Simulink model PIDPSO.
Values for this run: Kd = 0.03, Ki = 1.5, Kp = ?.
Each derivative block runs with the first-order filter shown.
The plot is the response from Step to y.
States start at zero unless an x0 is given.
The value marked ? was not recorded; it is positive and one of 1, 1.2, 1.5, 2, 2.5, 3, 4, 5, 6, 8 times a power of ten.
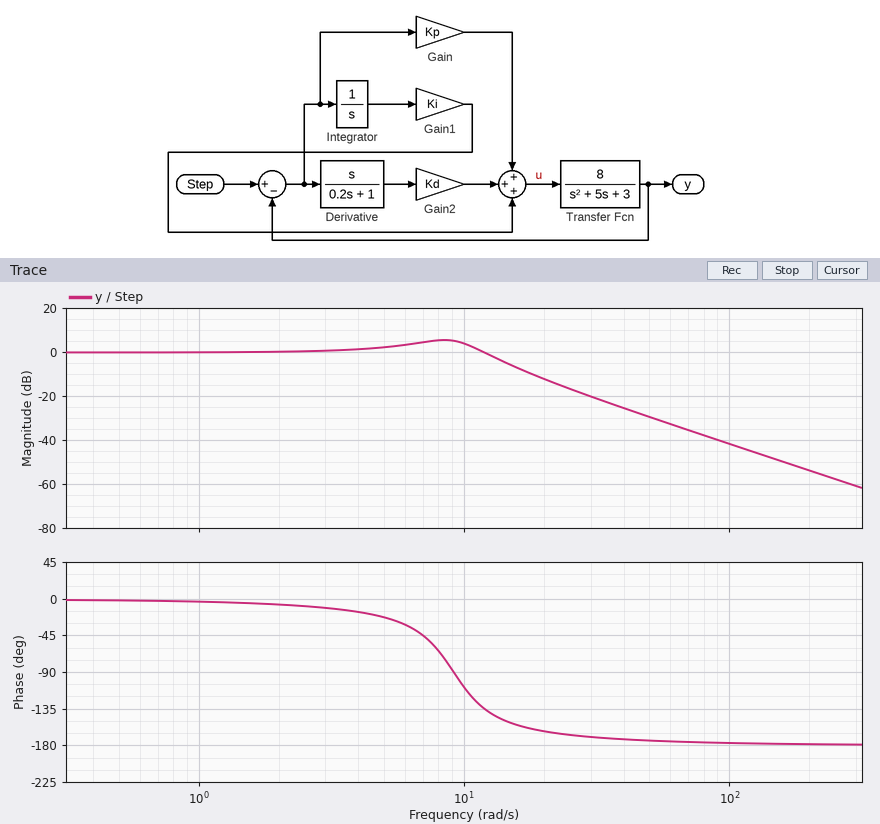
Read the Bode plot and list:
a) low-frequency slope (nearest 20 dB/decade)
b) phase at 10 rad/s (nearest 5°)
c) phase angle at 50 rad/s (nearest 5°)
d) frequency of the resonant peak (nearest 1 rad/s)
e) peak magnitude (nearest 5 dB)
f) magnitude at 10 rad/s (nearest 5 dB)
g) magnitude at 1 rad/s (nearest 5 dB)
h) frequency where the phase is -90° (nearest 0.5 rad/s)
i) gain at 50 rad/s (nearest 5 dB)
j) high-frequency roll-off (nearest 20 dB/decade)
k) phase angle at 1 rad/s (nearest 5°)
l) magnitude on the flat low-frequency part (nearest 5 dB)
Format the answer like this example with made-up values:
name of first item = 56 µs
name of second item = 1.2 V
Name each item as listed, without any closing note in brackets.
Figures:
low-frequency slope = 0 dB/decade
phase at 10 rad/s = -110°
phase angle at 50 rad/s = -175°
frequency of the resonant peak = 8 rad/s
peak magnitude = 5 dB
magnitude at 10 rad/s = 5 dB
magnitude at 1 rad/s = 0 dB
frequency where the phase is -90° = 9.0 rad/s
gain at 50 rad/s = -30 dB
high-frequency roll-off = -40 dB/decade
phase angle at 1 rad/s = -5°
magnitude on the flat low-frequency part = 0 dB
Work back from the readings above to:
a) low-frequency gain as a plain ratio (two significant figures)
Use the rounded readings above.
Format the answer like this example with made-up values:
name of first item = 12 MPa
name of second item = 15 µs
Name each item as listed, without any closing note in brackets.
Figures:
low-frequency gain as a plain ratio = 1.0
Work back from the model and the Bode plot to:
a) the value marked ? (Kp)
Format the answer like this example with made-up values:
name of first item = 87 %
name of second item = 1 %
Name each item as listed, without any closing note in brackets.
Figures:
the value marked ? = 10
